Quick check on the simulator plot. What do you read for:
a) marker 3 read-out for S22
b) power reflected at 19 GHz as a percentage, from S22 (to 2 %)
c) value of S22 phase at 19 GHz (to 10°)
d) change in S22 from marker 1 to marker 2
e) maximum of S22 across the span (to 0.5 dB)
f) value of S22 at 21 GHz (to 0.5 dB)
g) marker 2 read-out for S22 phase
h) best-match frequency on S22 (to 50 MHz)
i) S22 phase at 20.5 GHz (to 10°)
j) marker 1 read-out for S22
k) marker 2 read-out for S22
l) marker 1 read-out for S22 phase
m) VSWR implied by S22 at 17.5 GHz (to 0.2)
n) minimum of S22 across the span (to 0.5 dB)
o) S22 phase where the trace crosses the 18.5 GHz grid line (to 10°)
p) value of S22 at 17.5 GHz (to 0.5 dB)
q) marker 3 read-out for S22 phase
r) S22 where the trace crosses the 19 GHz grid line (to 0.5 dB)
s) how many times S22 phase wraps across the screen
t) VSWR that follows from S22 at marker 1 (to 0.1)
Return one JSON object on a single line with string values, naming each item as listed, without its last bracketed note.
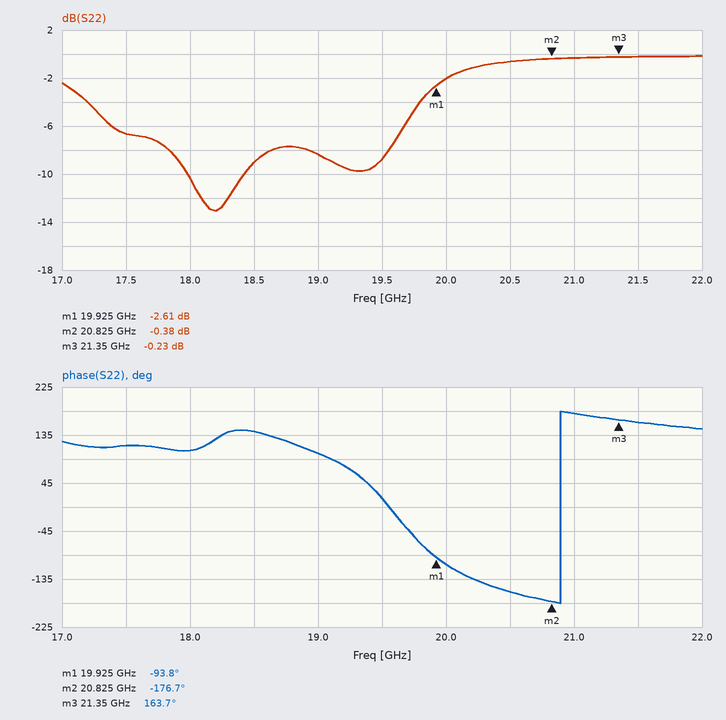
{"marker 3 read-out for S22": "-0.23 dB", "power reflected at 19 GHz as a percentage, from S22": "14 %", "value of S22 phase at 19 GHz": "100°", "change in S22 from marker 1 to marker 2": "2.23 dB", "maximum of S22 across the span": "0.0 dB", "value of S22 at 21 GHz": "-0.5 dB", "marker 2 read-out for S22 phase": "-176.7°", "best-match frequency on S22": "18.20 GHz", "S22 phase at 20.5 GHz": "-160°", "marker 1 read-out for S22": "-2.61 dB", "marker 2 read-out for S22": "-0.38 dB", "marker 1 read-out for S22 phase": "-93.8°", "VSWR implied by S22 at 17.5 GHz": "2.8", "minimum of S22 across the span": "-13.0 dB", "S22 phase where the trace crosses the 18.5 GHz grid line": "140°", "value of S22 at 17.5 GHz": "-6.5 dB", "marker 3 read-out for S22 phase": "163.7°", "S22 where the trace crosses the 19 GHz grid line": "-8.5 dB", "how many times S22 phase wraps across the screen": "1", "VSWR that follows from S22 at marker 1": "6.7"}
